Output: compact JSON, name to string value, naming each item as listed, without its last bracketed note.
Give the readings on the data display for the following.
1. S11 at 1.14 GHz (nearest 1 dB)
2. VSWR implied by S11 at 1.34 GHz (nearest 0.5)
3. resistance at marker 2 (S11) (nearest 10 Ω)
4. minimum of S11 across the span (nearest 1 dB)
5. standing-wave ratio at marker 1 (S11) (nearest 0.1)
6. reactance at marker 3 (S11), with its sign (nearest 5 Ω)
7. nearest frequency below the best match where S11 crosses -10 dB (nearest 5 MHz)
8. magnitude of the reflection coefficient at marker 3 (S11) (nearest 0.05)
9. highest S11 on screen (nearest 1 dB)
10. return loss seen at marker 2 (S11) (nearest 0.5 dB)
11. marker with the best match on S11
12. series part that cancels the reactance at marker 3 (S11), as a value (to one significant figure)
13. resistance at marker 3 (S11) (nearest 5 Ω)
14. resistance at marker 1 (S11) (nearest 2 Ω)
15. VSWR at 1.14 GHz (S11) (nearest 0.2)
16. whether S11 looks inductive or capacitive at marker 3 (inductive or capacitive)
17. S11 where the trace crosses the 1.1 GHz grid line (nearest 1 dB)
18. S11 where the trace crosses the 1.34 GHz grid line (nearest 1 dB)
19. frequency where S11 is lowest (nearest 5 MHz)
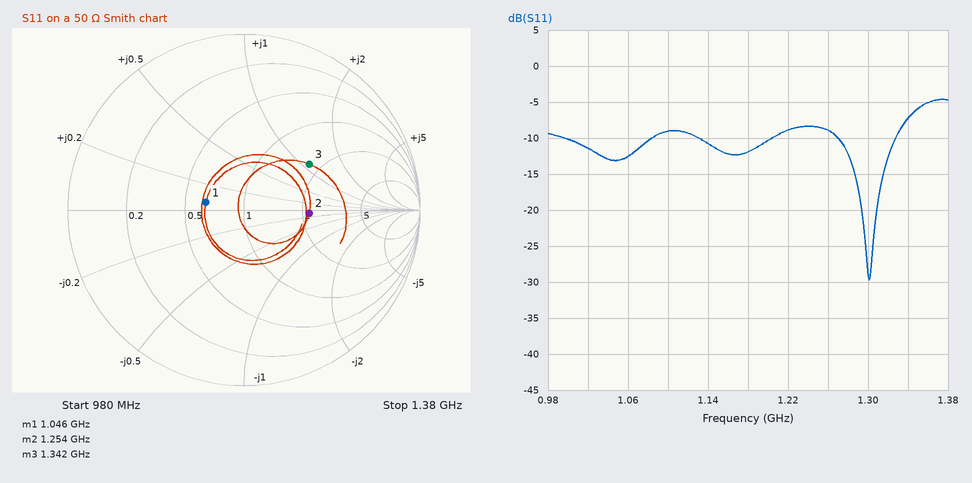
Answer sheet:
{"S11 at 1.14 GHz": "-11 dB", "VSWR implied by S11 at 1.34 GHz": "2.5", "resistance at marker 2 (S11)": "110 Ω", "minimum of S11 across the span": "-30 dB", "standing-wave ratio at marker 1 (S11)": "1.6", "reactance at marker 3 (S11), with its sign": "+55 Ω", "nearest frequency below the best match where S11 crosses -10 dB": "1.270 GHz", "magnitude of the reflection coefficient at marker 3 (S11)": "0.45", "highest S11 on screen": "-5 dB", "return loss seen at marker 2 (S11)": "8.5 dB", "marker with the best match on S11": "marker 1", "series part that cancels the reactance at marker 3 (S11), as a value": "2 pF", "resistance at marker 3 (S11)": "85 Ω", "resistance at marker 1 (S11)": "32 Ω", "VSWR at 1.14 GHz (S11)": "1.8", "whether S11 looks inductive or capacitive at marker 3": "inductive", "S11 where the trace crosses the 1.1 GHz grid line": "-9 dB", "S11 where the trace crosses the 1.34 GHz grid line": "-7 dB", "frequency where S11 is lowest": "1.300 GHz"}
